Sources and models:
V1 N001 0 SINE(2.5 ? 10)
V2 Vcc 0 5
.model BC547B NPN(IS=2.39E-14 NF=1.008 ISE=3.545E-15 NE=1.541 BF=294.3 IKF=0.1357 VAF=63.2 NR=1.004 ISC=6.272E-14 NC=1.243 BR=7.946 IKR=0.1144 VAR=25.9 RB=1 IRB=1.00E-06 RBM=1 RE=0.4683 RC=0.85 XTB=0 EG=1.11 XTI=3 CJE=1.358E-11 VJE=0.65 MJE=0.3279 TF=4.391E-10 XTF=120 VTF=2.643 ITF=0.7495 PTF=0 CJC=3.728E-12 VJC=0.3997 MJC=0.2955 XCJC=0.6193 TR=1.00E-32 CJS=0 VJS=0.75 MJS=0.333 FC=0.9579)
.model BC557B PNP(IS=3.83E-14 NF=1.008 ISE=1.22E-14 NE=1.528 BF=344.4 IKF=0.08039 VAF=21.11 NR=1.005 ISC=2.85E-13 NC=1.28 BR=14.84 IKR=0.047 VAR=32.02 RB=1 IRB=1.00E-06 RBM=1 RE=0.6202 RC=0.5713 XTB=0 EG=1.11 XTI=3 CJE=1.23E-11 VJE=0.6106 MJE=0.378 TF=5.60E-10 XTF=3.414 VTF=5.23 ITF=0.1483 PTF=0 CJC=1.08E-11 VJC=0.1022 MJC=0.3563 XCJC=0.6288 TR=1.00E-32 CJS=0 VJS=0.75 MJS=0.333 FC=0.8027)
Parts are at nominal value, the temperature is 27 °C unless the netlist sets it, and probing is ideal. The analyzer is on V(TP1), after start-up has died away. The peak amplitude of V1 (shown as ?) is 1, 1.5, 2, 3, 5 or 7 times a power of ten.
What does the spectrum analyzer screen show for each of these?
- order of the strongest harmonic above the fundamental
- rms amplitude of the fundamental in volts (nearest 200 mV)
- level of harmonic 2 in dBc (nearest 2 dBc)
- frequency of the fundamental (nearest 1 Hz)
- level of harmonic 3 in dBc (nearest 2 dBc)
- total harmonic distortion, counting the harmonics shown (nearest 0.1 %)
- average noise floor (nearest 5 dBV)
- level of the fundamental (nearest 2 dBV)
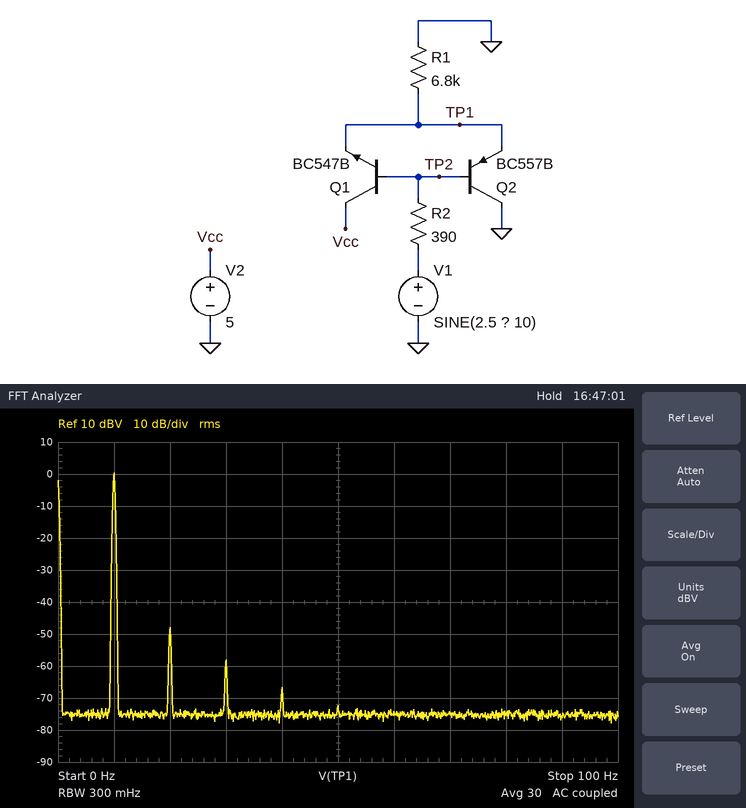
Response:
2
1.0 V
-48 dBc
10 Hz
-58 dBc
0.4 %
-75 dBV
0 dBV
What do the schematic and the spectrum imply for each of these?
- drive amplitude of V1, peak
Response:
1.5 V
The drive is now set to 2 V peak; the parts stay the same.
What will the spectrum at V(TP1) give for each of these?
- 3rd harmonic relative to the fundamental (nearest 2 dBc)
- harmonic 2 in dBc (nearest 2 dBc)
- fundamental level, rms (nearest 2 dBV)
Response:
-44 dBc
-40 dBc
2 dBV
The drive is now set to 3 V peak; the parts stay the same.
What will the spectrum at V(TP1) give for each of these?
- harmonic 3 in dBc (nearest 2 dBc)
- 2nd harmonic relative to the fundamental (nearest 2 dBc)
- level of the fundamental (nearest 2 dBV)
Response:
-24 dBc
-20 dBc
6 dBV
